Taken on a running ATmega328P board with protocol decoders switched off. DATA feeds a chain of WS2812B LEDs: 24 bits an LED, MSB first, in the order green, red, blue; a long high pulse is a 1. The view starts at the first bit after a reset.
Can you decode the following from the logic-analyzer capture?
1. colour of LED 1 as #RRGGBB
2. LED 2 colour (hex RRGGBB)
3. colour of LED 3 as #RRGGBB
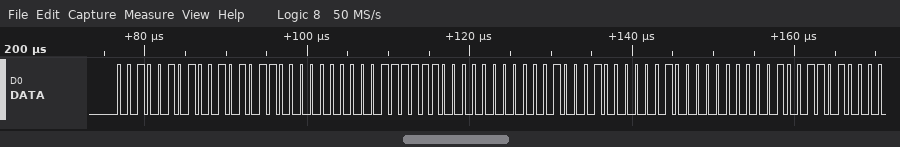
#2B2500
#003F11
#00024D
